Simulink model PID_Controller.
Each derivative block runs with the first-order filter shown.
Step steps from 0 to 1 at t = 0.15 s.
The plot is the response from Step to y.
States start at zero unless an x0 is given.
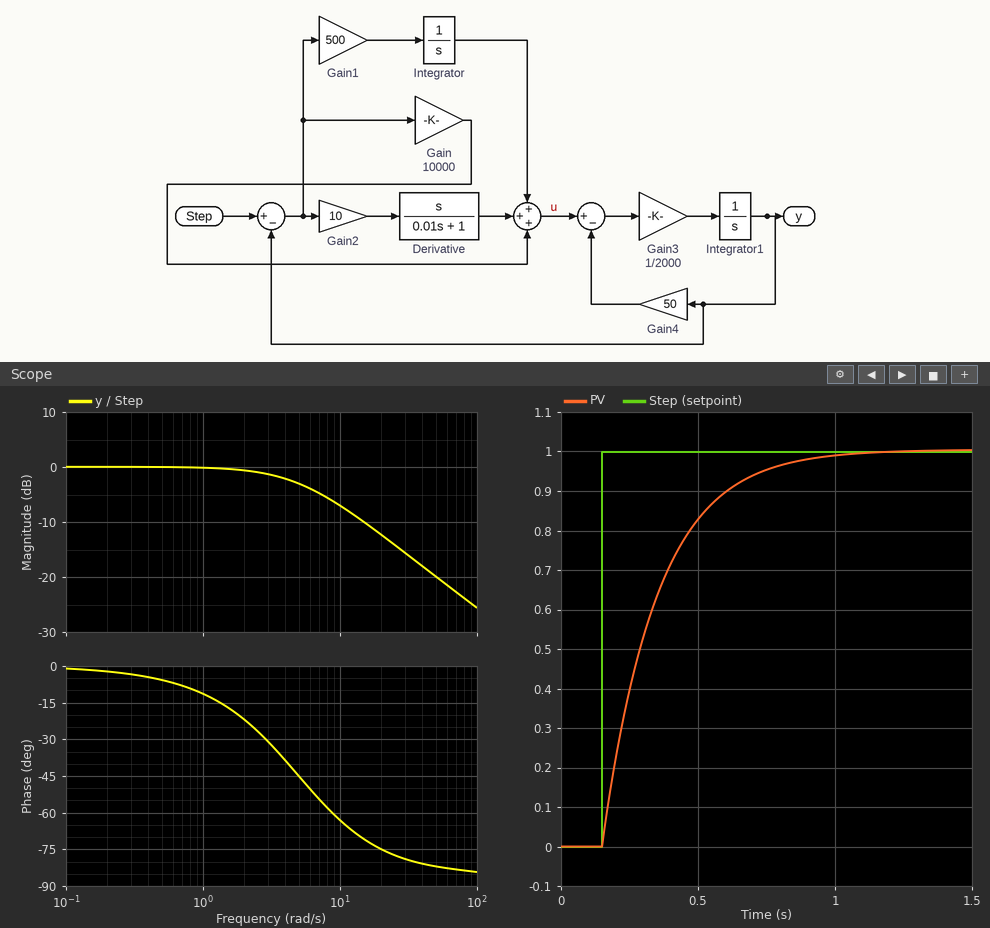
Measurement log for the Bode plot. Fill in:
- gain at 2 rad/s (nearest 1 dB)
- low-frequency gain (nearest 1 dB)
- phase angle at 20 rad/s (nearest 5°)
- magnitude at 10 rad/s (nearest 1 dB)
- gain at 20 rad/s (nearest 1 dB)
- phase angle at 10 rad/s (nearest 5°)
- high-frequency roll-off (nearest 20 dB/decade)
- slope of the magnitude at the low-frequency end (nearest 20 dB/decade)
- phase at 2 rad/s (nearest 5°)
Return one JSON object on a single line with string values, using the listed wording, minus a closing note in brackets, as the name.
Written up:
{"gain at 2 rad/s": "-1 dB", "low-frequency gain": "0 dB", "phase angle at 20 rad/s": "-75°", "magnitude at 10 rad/s": "-7 dB", "gain at 20 rad/s": "-12 dB", "phase angle at 10 rad/s": "-65°", "high-frequency roll-off": "-20 dB/decade", "slope of the magnitude at the low-frequency end": "0 dB/decade", "phase at 2 rad/s": "-20°"}
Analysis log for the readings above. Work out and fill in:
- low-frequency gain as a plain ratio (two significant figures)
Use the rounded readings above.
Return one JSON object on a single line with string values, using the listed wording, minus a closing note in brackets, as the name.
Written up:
{"low-frequency gain as a plain ratio": "1.0"}
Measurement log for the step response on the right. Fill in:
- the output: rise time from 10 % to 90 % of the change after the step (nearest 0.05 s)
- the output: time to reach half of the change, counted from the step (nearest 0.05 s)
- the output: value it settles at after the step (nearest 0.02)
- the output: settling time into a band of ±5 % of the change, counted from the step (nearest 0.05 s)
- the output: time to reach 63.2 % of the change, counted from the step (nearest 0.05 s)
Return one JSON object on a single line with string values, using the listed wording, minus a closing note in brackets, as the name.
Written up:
{"the output: rise time from 10 % to 90 % of the change after the step": "0.45 s", "the output: time to reach half of the change, counted from the step": "0.15 s", "the output: value it settles at after the step": "1.00", "the output: settling time into a band of ±5 % of the change, counted from the step": "0.60 s", "the output: time to reach 63.2 % of the change, counted from the step": "0.20 s"}
